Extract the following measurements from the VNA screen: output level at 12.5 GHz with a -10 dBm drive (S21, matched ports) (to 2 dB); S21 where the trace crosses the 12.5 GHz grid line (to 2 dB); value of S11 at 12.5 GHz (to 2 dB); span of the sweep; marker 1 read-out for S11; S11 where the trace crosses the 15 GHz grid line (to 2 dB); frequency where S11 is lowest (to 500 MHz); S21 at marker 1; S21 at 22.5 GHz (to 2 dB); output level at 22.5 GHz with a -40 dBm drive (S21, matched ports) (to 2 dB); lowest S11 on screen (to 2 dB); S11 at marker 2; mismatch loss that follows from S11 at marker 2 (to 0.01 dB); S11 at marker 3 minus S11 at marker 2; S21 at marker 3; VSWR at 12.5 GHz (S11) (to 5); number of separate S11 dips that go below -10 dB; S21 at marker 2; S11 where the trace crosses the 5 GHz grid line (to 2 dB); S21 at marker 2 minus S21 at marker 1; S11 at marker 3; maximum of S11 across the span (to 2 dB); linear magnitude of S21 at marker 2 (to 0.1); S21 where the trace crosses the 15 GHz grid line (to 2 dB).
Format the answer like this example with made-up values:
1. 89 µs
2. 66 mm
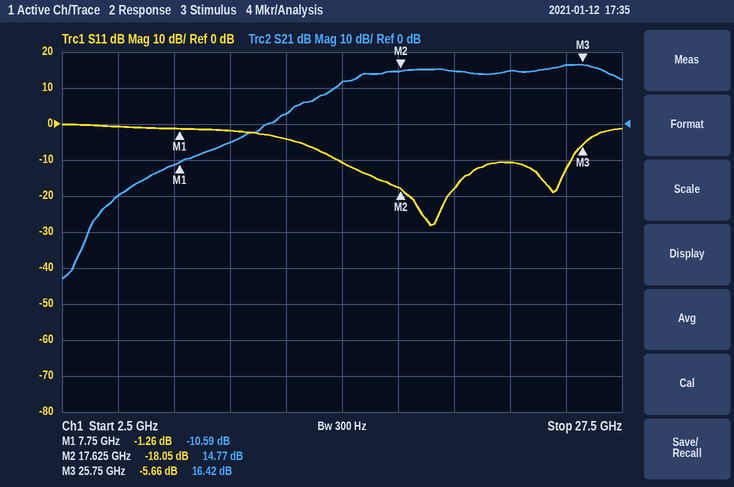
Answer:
1. -8 dBm
2. 2 dB
3. -4 dB
4. 25 GHz
5. -1.26 dB
6. -10 dB
7. 19.0 GHz
8. -10.59 dB
9. 14 dB
10. -26 dBm
11. -28 dB
12. -18.05 dB
13. 0.07 dB
14. 12.39 dB
15. 16.42 dB
16. 5
17. 2
18. 14.77 dB
19. 0 dB
20. 25.36 dB
21. -5.66 dB
22. 0 dB
23. 5.5
24. 12 dB
